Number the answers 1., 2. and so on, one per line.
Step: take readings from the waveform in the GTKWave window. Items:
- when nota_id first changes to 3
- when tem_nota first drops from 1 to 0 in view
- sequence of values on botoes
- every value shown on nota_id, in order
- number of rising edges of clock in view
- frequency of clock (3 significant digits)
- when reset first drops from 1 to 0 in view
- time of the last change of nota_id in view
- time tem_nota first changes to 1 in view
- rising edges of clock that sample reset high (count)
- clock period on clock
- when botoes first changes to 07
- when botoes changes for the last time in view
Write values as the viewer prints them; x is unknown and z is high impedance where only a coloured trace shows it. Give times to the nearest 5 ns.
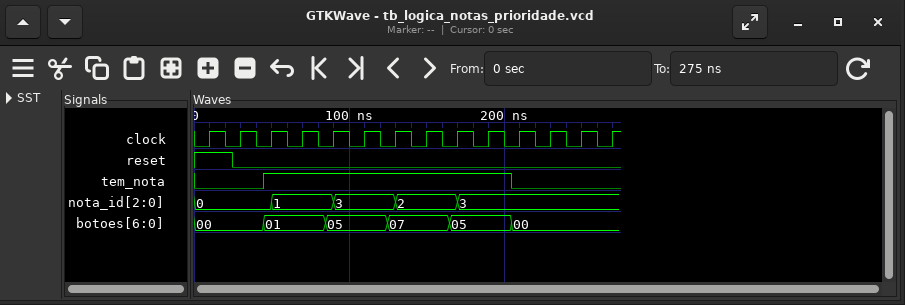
1. 90 ns
2. 205 ns
3. 00, 01, 05, 07, 05, 00
4. 0, 1, 3, 2, 3
5. 14
6. 50.0 MHz
7. 25 ns
8. 170 ns
9. 45 ns
10. 1
11. 20 ns
12. 125 ns
13. 205 ns
